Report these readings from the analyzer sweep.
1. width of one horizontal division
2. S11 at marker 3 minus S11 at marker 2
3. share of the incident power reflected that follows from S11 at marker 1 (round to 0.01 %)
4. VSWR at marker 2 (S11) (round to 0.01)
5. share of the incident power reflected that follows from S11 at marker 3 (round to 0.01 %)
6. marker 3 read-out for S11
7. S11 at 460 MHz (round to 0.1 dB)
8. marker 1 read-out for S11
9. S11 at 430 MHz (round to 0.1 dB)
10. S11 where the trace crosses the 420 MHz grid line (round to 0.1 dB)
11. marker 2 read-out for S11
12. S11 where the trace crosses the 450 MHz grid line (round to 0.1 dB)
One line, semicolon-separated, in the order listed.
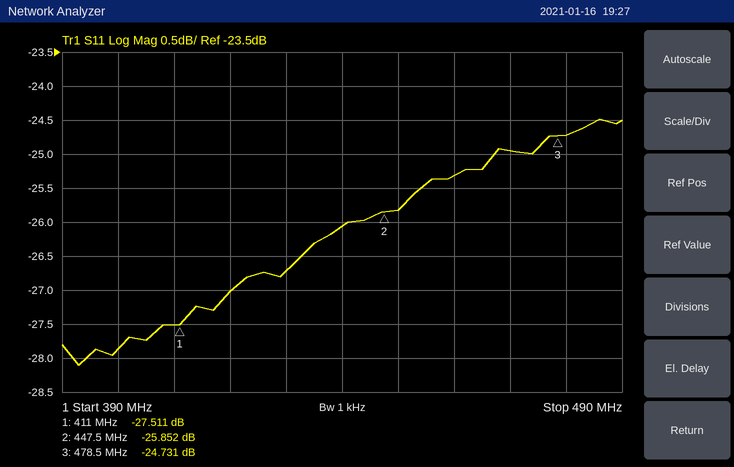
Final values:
10 MHz; 1.121 dB; 0.18 %; 1.11; 0.34 %; -24.731 dB; -25.3 dB; -27.511 dB; -26.7 dB; -27.0 dB; -25.852 dB; -25.8 dB
